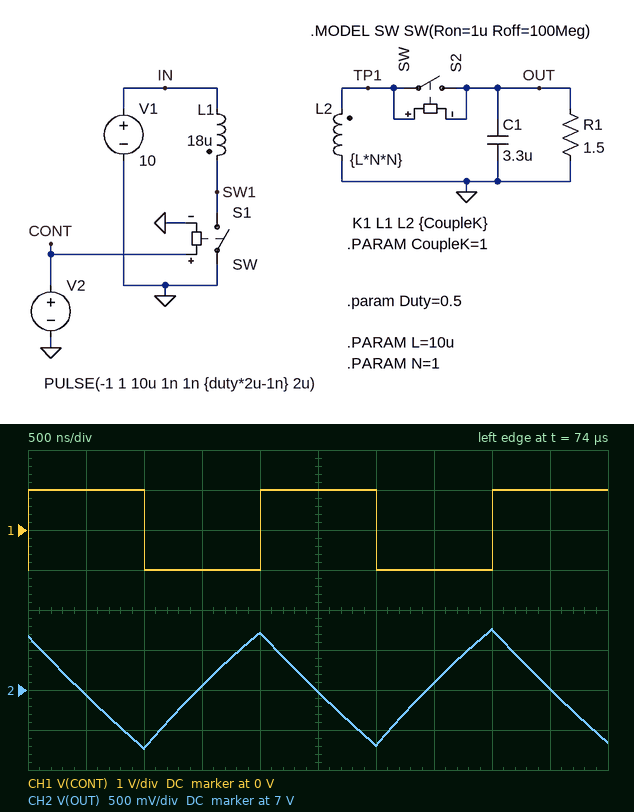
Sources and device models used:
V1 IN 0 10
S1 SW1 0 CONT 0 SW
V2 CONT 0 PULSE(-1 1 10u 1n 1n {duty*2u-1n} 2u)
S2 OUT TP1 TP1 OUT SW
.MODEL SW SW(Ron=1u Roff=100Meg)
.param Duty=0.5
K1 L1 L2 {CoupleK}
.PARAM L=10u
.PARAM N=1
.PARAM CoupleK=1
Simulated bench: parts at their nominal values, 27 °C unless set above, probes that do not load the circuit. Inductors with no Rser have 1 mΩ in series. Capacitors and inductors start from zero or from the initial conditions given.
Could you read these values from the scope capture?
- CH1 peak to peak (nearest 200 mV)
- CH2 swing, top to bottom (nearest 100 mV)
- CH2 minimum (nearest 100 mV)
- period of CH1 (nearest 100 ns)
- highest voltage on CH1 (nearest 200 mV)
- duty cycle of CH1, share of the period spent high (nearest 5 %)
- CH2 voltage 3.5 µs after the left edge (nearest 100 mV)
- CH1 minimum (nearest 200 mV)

2.0 V
1.5 V
6.3 V
2.0 µs
1.0 V
50 %
7.1 V
-1.0 V
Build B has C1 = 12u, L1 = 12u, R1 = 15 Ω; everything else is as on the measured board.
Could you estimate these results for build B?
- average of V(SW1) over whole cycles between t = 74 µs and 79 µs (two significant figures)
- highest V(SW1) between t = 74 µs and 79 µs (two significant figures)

14 V
28 V
